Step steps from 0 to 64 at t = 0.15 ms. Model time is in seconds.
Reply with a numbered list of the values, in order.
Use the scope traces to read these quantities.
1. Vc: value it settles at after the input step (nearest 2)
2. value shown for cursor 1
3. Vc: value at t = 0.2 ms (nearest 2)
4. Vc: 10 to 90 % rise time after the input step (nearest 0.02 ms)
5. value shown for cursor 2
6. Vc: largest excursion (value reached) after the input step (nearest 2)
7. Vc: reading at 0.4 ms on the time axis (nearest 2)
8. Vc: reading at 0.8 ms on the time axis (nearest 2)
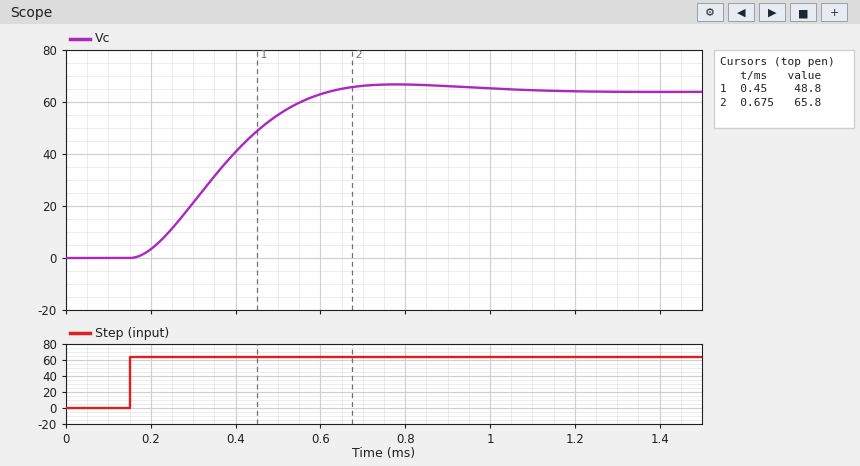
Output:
1. 64
2. 48.8
3. 4
4. 0.30 ms
5. 65.8
6. 66
7. 40
8. 66
